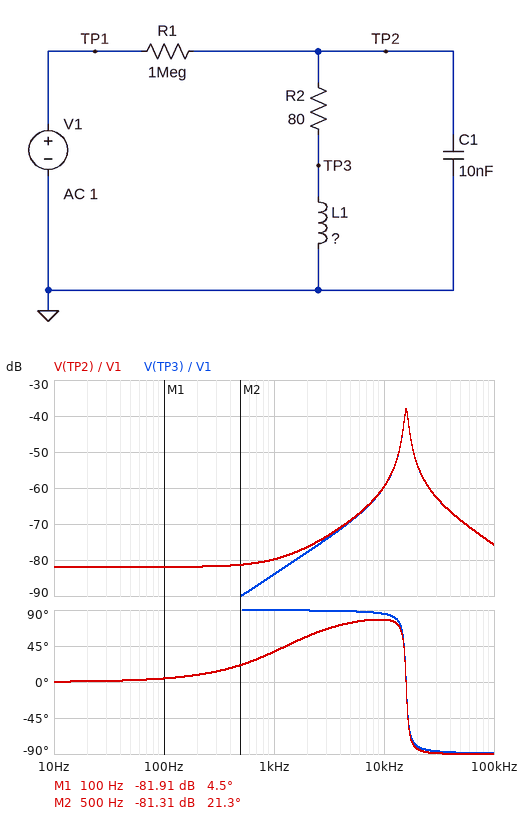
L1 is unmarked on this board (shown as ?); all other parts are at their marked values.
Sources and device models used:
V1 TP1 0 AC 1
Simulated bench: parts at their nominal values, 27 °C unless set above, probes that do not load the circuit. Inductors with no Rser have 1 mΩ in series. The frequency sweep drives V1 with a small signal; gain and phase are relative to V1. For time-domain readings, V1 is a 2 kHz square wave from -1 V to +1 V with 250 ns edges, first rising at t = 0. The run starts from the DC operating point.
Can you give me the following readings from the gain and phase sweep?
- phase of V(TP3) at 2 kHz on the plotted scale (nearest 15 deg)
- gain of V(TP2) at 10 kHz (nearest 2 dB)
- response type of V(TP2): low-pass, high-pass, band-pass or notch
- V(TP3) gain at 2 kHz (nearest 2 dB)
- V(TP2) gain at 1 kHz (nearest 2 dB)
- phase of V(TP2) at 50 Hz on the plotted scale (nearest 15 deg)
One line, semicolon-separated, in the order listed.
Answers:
90 deg; -60 dB; band-pass; -78 dB; -80 dB; 0 deg
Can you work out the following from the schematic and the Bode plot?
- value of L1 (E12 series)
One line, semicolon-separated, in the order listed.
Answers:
10 mH
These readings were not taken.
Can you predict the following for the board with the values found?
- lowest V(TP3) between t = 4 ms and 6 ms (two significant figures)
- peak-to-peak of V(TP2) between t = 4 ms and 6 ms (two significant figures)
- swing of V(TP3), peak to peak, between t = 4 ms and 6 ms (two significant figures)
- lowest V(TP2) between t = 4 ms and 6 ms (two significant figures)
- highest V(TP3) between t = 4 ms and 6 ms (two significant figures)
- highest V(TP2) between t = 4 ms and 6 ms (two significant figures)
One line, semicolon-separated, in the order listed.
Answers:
-1.4 mV; 2.9 mV; 2.8 mV; -1.5 mV; 1.4 mV; 1.5 mV
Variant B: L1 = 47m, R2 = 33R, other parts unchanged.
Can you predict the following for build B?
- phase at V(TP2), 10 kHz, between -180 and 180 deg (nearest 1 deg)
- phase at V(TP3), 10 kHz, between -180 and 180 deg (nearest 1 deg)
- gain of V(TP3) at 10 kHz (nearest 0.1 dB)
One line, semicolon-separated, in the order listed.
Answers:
-89 deg; -88 deg; -49.2 dB
